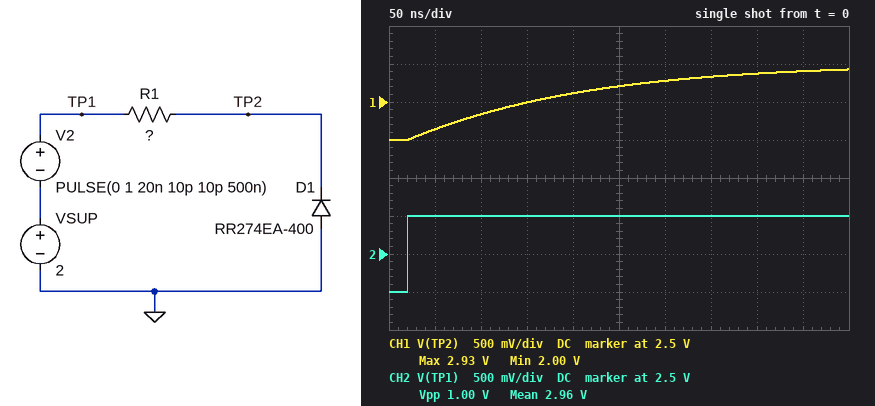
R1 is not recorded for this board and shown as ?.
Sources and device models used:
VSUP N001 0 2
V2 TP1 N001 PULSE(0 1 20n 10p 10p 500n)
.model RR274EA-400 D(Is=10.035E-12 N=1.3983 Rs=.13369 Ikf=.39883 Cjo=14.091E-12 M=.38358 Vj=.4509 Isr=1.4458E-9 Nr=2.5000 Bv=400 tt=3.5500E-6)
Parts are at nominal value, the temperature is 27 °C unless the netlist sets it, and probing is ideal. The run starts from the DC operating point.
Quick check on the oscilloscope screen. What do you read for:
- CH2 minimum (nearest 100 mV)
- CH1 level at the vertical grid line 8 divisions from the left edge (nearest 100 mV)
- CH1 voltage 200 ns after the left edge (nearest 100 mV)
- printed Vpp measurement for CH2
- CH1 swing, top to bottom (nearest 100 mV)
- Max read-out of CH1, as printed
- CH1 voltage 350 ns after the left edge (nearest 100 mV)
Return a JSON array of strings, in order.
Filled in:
["2.0 V", "2.9 V", "2.6 V", "1.00 V", "900 mV", "2.93 V", "2.8 V"]
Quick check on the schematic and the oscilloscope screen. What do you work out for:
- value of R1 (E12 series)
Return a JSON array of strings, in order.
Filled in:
["27 kΩ"]
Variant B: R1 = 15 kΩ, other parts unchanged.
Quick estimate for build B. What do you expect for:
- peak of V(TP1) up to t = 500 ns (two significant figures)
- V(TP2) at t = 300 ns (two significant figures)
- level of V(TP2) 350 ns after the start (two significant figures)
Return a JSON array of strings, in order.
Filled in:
["3.0 V", "2.9 V", "3.0 V"]
